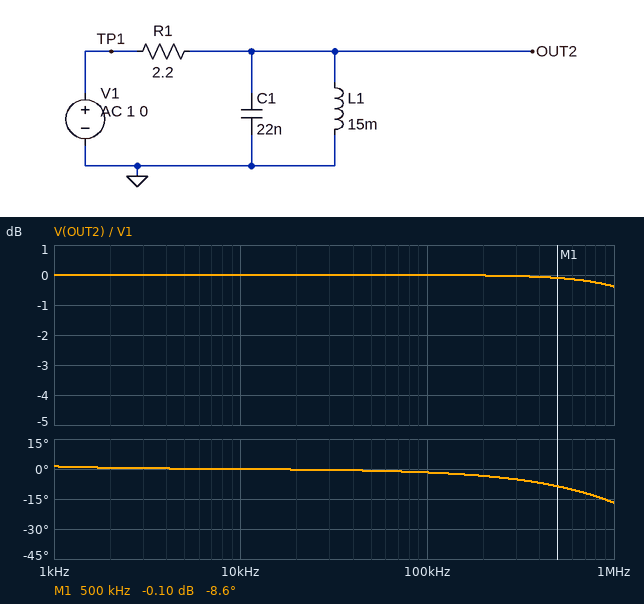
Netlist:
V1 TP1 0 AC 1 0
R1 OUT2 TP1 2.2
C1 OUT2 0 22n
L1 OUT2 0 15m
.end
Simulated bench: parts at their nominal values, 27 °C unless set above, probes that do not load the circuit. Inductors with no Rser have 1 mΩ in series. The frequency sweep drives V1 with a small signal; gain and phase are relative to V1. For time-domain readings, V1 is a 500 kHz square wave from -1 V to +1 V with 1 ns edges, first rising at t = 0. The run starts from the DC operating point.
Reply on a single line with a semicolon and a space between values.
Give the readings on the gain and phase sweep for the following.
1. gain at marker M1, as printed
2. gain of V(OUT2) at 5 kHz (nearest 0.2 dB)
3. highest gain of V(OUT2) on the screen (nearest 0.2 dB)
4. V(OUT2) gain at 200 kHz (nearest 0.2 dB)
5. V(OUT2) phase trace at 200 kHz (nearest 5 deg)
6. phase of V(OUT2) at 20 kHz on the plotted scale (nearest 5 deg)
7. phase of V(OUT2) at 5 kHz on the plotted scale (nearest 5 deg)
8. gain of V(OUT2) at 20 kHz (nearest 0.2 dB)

-0.10 dB; 0 dB; 0 dB; 0 dB; -5 deg; 0 deg; 0 deg; 0 dB
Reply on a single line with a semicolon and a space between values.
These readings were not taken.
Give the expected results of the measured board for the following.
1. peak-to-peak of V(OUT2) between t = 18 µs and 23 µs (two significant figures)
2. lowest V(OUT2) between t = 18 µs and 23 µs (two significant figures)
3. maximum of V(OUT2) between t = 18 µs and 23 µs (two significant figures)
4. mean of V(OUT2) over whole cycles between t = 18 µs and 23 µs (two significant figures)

2.0 V; -3.7 mV; 2.0 V; 1.0 V
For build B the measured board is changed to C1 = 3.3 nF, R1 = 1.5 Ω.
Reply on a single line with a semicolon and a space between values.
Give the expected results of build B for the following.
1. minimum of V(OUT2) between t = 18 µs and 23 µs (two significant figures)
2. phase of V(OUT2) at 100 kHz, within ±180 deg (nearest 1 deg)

-2.9 mV; 0 deg
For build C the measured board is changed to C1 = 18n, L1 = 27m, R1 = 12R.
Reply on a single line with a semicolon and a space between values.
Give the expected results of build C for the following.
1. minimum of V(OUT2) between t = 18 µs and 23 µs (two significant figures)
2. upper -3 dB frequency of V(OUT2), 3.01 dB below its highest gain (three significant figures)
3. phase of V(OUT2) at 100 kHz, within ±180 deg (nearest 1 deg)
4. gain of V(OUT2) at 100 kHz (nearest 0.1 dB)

9.6 mV; 737 kHz; -8 deg; -0.1 dB
